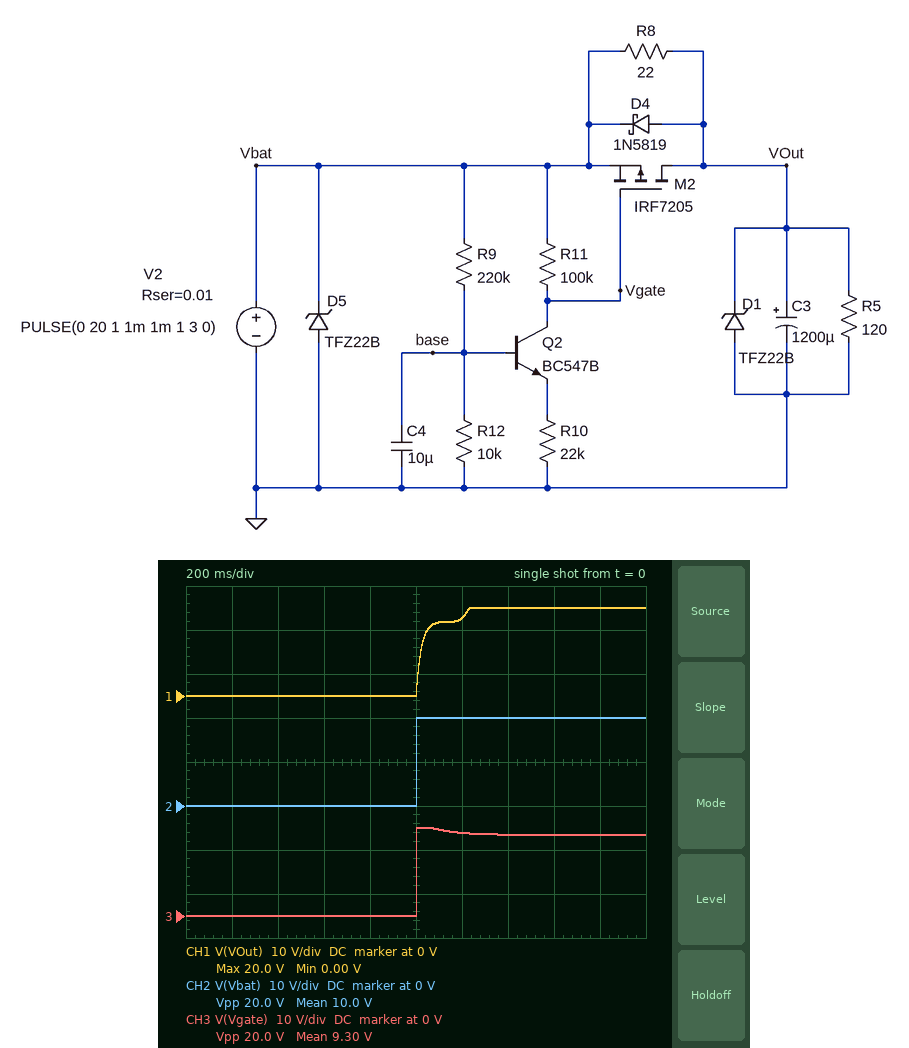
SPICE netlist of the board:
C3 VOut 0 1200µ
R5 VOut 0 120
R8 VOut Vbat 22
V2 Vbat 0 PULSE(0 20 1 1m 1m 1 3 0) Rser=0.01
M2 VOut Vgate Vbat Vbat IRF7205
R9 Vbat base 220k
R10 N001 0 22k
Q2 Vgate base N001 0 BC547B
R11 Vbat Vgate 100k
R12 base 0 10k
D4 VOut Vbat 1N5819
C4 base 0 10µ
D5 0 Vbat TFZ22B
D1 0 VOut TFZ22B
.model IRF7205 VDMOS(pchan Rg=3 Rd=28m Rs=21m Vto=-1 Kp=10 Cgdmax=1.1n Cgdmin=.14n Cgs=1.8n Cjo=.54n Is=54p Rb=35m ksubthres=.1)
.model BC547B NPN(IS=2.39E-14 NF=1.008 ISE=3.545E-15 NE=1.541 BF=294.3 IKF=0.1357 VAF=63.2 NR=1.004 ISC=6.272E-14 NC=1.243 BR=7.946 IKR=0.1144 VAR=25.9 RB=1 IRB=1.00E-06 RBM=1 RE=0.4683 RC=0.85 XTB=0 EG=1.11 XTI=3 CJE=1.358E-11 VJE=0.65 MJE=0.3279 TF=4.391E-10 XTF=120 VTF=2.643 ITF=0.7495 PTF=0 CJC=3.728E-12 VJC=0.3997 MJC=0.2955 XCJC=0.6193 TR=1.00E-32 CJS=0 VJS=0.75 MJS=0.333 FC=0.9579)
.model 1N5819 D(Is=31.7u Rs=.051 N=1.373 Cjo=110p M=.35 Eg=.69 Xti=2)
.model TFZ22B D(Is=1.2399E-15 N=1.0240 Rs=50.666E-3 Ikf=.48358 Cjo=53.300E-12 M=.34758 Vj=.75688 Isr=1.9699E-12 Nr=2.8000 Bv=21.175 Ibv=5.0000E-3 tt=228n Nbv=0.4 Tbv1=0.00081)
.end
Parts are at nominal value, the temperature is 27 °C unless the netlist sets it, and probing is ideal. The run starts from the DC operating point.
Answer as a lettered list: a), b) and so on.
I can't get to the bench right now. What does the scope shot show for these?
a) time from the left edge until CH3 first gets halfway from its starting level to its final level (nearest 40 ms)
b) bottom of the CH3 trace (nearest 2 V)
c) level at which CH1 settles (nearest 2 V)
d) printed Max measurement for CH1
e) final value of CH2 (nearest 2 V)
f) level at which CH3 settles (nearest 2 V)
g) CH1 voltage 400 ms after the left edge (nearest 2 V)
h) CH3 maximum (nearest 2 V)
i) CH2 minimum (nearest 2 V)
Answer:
a) 1.00 s
b) 0 V
c) 20 V
d) 20.0 V
e) 20 V
f) 18 V
g) 0 V
h) 20 V
i) 0 V
